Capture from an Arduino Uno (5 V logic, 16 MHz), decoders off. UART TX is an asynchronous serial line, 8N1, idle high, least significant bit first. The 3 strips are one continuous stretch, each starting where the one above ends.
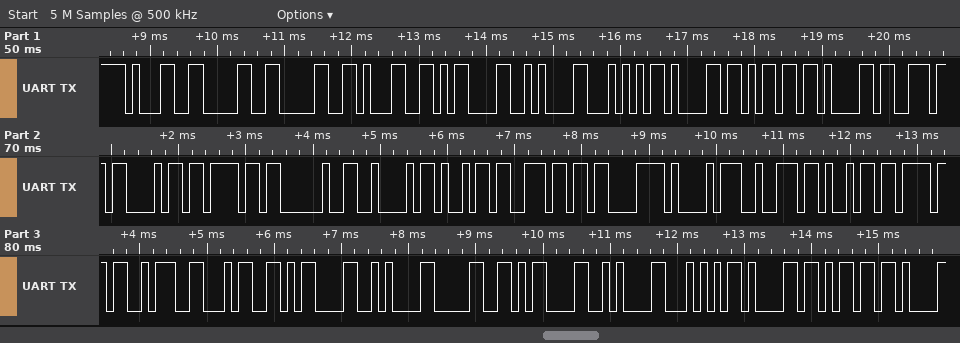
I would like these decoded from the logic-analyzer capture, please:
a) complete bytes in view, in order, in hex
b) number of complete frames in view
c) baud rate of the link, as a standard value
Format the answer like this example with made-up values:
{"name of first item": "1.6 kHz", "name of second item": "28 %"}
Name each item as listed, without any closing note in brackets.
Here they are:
{"complete bytes in view, in order, in hex": "0x31 0x30 0x30 0x31 0x0D 0x0A 0x54 0x61 0x6D 0x61 0x6E 0x68 0x6F 0x20 0x42 0x69 0x6E 0xC3 0xA1 0x72 0x69 0x6F 0x3A 0x34 0x0D 0x0A 0x30 0x0D 0x0A 0x54 0x61 0x6D", "number of complete frames in view": "32", "baud rate of the link, as a standard value": "9600 baud"}
